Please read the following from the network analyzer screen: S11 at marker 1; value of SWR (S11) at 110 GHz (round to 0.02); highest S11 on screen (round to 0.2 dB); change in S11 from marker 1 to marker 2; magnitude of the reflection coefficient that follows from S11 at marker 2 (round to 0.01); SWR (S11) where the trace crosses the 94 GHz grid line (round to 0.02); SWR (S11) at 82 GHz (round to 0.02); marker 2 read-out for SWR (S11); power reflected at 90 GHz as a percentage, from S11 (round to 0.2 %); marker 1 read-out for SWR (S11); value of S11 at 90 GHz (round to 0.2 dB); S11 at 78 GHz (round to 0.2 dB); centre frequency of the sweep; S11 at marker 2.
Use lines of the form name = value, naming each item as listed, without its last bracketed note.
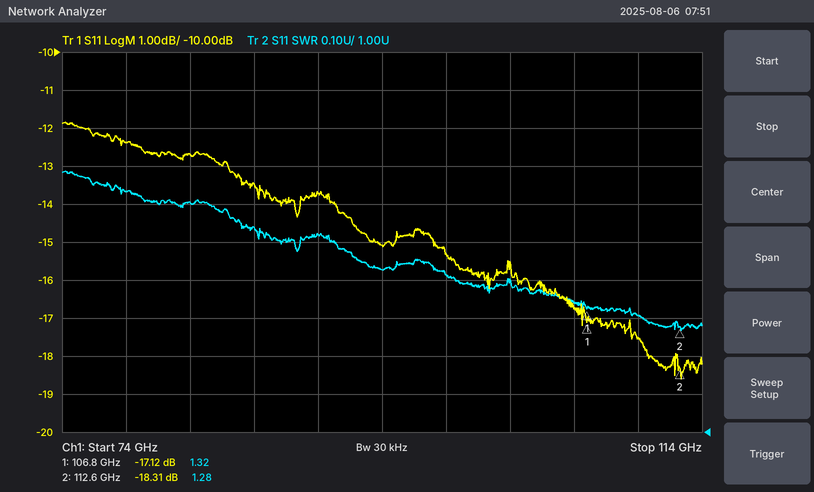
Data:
S11 at marker 1 = -17.12 dB
value of SWR (S11) at 110 GHz = 1.30
highest S11 on screen = -11.8 dB
change in S11 from marker 1 to marker 2 = -1.19 dB
magnitude of the reflection coefficient that follows from S11 at marker 2 = 0.12
SWR (S11) where the trace crosses the 94 GHz grid line = 1.42
SWR (S11) at 82 GHz = 1.60
marker 2 read-out for SWR = 1.28
power reflected at 90 GHz as a percentage, from S11 = 4.2 %
marker 1 read-out for SWR = 1.32
value of S11 at 90 GHz = -13.8 dB
S11 at 78 GHz = -12.4 dB
centre frequency of the sweep = 94 GHz
S11 at marker 2 = -18.31 dB
